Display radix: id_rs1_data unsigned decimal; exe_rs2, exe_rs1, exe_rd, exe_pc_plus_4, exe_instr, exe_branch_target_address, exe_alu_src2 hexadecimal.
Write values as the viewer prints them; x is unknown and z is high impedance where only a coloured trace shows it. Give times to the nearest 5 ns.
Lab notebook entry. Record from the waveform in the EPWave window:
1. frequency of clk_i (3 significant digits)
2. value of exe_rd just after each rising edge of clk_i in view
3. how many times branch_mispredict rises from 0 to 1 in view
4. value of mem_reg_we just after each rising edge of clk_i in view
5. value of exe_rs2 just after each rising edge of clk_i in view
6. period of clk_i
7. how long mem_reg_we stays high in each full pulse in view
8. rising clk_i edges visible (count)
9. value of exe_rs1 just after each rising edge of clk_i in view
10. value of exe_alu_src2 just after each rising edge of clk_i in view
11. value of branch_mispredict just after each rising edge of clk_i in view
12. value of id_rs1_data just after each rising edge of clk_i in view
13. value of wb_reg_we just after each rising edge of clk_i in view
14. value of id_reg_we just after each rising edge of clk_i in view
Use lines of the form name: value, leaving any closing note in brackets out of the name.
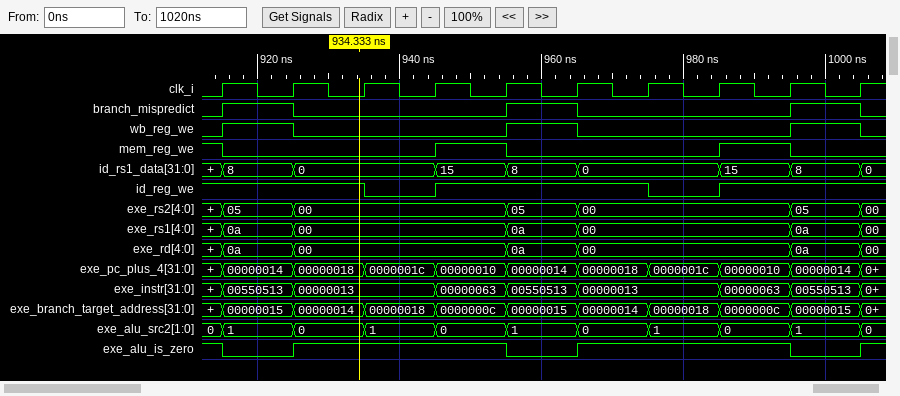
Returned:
frequency of clk_i: 100 MHz
value of exe_rd just after each rising edge of clk_i in view: 0a, 00, 00, 00, 0a, 00, 00, 00, 0a, 00
how many times branch_mispredict rises from 0 to 1 in view: 3
value of mem_reg_we just after each rising edge of clk_i in view: 0 0 0 1 0 0 0 1 0 0
value of exe_rs2 just after each rising edge of clk_i in view: 05, 00, 00, 00, 05, 00, 00, 00, 05, 00
period of clk_i: 10 ns
how long mem_reg_we stays high in each full pulse in view: 10 ns, 10 ns
rising clk_i edges visible: 10
value of exe_rs1 just after each rising edge of clk_i in view: 0a, 00, 00, 00, 0a, 00, 00, 00, 0a, 00
value of exe_alu_src2 just after each rising edge of clk_i in view: 1, 0, 1, 0, 1, 0, 1, 0, 1, 0
value of branch_mispredict just after each rising edge of clk_i in view: 1 0 0 0 1 0 0 0 1 0
value of id_rs1_data just after each rising edge of clk_i in view: 8, 0, 0, 15, 8, 0, 0, 15, 8, 0
value of wb_reg_we just after each rising edge of clk_i in view: 1 0 0 0 1 0 0 0 1 0
value of id_reg_we just after each rising edge of clk_i in view: 1 1 0 1 1 1 0 1 1 1
